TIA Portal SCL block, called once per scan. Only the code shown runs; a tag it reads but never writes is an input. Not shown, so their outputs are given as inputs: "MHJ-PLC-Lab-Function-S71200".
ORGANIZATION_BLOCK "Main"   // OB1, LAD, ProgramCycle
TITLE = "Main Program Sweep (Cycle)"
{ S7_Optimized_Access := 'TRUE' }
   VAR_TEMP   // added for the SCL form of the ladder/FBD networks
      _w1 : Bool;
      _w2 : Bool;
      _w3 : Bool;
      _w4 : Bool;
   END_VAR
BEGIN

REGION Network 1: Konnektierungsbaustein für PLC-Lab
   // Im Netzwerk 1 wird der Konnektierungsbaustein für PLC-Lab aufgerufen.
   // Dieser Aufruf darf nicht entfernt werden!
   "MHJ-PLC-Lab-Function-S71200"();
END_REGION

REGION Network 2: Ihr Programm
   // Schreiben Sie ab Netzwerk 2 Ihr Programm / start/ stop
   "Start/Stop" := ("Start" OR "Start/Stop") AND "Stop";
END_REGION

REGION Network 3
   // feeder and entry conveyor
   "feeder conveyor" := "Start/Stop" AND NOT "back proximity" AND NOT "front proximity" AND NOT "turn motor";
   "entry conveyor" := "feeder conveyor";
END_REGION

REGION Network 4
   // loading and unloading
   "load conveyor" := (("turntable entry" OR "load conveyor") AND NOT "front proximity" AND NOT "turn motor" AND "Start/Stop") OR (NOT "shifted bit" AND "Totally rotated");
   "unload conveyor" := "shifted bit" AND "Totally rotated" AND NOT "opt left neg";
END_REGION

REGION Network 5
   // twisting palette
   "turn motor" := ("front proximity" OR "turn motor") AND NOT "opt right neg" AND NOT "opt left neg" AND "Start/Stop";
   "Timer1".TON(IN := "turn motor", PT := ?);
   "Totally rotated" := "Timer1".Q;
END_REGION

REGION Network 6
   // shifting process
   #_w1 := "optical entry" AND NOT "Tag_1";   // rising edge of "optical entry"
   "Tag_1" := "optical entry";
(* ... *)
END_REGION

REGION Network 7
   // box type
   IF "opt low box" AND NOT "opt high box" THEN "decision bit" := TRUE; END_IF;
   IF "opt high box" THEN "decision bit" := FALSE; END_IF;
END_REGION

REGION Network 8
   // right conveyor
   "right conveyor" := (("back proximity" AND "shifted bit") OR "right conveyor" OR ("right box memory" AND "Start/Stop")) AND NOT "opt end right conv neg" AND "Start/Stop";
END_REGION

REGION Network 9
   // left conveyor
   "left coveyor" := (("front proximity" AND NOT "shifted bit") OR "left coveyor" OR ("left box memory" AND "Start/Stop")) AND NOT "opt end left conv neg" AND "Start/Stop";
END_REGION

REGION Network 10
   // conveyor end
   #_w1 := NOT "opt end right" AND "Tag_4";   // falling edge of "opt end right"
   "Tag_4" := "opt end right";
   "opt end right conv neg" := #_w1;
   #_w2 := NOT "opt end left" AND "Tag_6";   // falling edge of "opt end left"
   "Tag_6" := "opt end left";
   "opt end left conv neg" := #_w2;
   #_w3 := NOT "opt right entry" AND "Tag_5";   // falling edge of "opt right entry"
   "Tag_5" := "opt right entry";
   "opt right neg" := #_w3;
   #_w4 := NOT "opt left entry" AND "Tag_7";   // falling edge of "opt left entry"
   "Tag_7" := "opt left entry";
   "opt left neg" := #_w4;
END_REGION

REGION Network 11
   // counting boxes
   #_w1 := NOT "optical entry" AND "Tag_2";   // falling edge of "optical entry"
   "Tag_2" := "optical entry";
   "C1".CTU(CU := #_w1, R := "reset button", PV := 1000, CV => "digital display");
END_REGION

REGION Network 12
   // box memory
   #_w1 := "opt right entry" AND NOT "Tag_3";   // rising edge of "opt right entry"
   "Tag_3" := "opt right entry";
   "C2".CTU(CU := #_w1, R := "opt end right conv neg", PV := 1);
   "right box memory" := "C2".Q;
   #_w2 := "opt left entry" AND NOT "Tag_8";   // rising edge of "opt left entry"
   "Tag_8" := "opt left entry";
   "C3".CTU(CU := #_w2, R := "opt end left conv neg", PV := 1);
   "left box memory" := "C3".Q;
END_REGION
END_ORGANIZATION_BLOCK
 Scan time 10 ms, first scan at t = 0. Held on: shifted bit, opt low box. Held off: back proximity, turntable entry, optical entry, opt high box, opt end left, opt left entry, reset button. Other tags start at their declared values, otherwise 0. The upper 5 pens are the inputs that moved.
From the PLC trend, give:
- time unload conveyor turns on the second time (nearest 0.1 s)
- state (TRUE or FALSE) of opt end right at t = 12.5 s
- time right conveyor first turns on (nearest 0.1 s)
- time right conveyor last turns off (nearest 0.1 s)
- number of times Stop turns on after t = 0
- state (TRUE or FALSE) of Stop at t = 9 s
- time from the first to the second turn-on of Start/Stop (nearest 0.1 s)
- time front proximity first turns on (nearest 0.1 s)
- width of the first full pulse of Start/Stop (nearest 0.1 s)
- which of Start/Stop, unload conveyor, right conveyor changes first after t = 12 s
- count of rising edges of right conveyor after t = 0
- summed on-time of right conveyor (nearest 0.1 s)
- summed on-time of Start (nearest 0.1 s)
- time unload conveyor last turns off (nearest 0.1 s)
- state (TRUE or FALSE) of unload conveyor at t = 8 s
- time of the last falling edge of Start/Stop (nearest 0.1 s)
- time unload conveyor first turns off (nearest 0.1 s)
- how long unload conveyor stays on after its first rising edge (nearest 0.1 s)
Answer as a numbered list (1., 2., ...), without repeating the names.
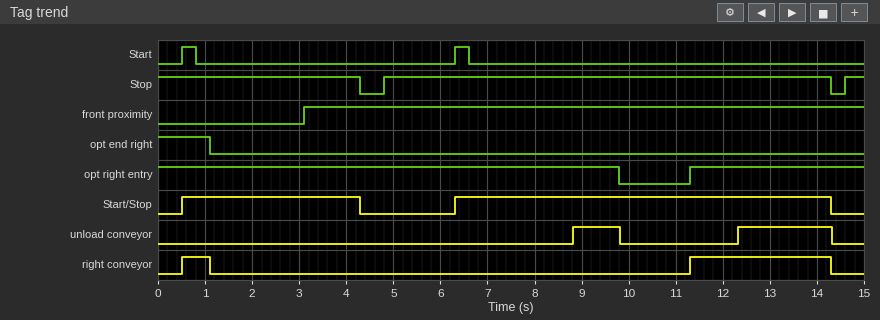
1. 12.3 s
2. FALSE
3. 0.5 s
4. 14.3 s
5. 2
6. TRUE
7. 5.8 s
8. 3.1 s
9. 3.8 s
10. unload conveyor
11. 2
12. 3.6 s
13. 0.6 s
14. 14.3 s
15. FALSE
16. 14.3 s
17. 9.8 s
18. 1.0 s
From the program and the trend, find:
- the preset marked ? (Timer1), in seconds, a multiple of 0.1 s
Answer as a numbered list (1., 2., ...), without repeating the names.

1. 2.5 s
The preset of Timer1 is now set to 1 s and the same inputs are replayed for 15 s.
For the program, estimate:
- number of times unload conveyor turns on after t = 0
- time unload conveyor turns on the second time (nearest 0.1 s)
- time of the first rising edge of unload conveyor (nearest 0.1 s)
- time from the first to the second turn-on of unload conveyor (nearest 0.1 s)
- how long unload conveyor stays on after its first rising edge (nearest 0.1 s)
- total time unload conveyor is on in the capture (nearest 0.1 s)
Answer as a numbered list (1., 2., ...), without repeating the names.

1. 3
2. 7.3 s
3. 4.1 s
4. 3.2 s
5. 0.2 s
6. 6.2 s
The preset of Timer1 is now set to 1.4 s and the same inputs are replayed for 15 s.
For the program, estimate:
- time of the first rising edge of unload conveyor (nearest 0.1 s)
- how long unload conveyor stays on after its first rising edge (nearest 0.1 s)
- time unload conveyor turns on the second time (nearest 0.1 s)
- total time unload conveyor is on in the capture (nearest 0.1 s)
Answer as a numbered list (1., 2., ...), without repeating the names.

1. 7.7 s
2. 2.1 s
3. 11.2 s
4. 5.2 s
